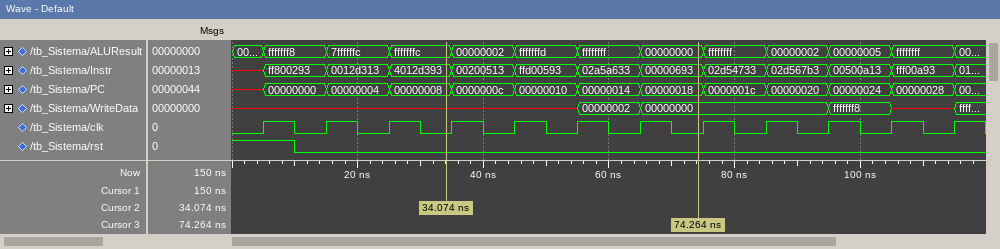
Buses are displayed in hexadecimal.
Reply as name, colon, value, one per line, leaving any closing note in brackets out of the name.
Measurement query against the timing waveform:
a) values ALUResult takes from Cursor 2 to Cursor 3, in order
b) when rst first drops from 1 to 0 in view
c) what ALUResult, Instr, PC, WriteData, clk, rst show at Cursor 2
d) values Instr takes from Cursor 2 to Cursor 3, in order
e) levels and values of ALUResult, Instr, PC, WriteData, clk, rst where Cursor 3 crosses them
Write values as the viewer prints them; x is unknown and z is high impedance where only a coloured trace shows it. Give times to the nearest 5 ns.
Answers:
values ALUResult takes from Cursor 2 to Cursor 3, in order: fffffffc, 00000002, fffffffd, ffffffff, 00000000
when rst first drops from 1 to 0 in view: 10 ns
what ALUResult, Instr, PC, WriteData, clk, rst show at Cursor 2: ALUResult=fffffffc, Instr=4012d393, PC=00000008, WriteData=x, clk=0, rst=0
values Instr takes from Cursor 2 to Cursor 3, in order: 4012d393, 00200513, ffd00593, 02a5a633, 00000693
levels and values of ALUResult, Instr, PC, WriteData, clk, rst where Cursor 3 crosses them: ALUResult=00000000, Instr=00000693, PC=00000018, WriteData=00000000, clk=0, rst=0
